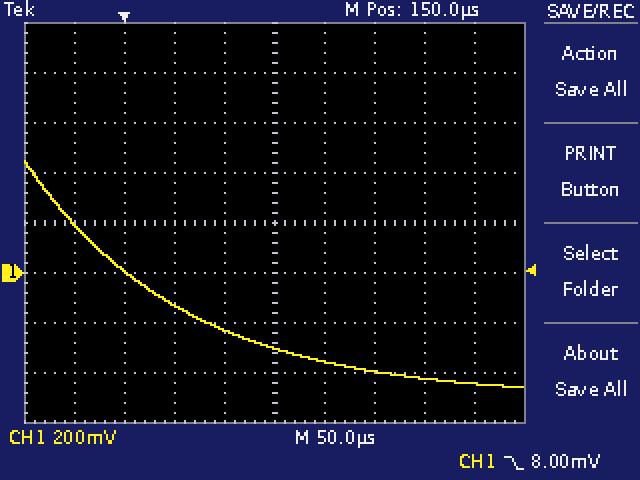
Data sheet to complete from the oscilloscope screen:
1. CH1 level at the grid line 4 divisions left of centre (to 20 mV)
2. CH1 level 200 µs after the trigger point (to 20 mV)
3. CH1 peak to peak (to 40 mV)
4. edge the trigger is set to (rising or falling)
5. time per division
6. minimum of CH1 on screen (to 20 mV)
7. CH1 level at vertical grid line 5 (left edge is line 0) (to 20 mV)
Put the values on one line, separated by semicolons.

200 mV; -360 mV; 920 mV; falling; 50 µs; -460 mV; -300 mV
